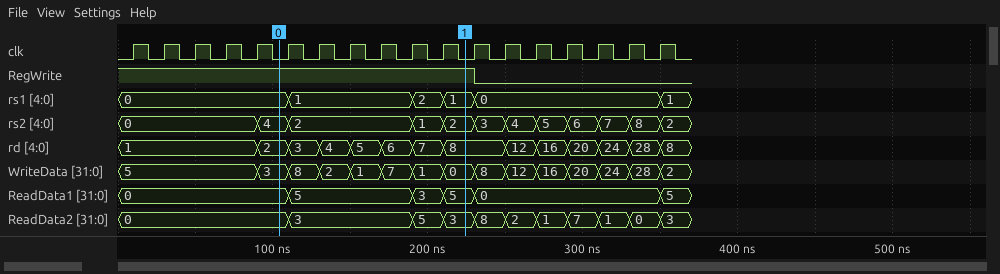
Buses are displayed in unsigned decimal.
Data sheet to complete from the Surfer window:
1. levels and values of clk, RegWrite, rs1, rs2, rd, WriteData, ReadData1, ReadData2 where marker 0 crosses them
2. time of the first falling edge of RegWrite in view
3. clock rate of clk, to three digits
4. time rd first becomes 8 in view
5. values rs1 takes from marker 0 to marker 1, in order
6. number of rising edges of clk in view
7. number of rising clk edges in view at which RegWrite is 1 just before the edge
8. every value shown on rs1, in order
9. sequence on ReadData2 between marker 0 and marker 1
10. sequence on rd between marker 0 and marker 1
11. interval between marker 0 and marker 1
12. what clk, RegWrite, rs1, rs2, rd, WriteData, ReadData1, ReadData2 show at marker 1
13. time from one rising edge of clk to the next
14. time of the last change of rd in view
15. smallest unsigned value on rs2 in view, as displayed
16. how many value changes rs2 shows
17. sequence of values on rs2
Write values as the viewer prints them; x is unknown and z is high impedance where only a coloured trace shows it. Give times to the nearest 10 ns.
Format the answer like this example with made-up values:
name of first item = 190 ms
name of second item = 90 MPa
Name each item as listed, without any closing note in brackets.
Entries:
levels and values of clk, RegWrite, rs1, rs2, rd, WriteData, ReadData1, ReadData2 where marker 0 crosses them = clk=0, RegWrite=1, rs1=0, rs2=4, rd=2, WriteData=3, ReadData1=0, ReadData2=0
time of the first falling edge of RegWrite in view = 230 ns
clock rate of clk, to three digits = 50.0 MHz
time rd first becomes 8 in view = 210 ns
values rs1 takes from marker 0 to marker 1, in order = 0, 1, 2, 1
number of rising edges of clk in view = 18
number of rising clk edges in view at which RegWrite is 1 just before the edge = 12
every value shown on rs1, in order = 0, 1, 2, 1, 0, 1
sequence on ReadData2 between marker 0 and marker 1 = 0, 3, 5, 3
sequence on rd between marker 0 and marker 1 = 2, 3, 4, 5, 6, 7, 8
interval between marker 0 and marker 1 = 120 ns
what clk, RegWrite, rs1, rs2, rd, WriteData, ReadData1, ReadData2 show at marker 1 = clk=0, RegWrite=1, rs1=1, rs2=2, rd=8, WriteData=0, ReadData1=5, ReadData2=3
time from one rising edge of clk to the next = 20 ns
time of the last change of rd in view = 350 ns
smallest unsigned value on rs2 in view, as displayed = 0
how many value changes rs2 shows = 11
sequence of values on rs2 = 0, 4, 2, 1, 2, 3, 4, 5, 6, 7, 8, 2
